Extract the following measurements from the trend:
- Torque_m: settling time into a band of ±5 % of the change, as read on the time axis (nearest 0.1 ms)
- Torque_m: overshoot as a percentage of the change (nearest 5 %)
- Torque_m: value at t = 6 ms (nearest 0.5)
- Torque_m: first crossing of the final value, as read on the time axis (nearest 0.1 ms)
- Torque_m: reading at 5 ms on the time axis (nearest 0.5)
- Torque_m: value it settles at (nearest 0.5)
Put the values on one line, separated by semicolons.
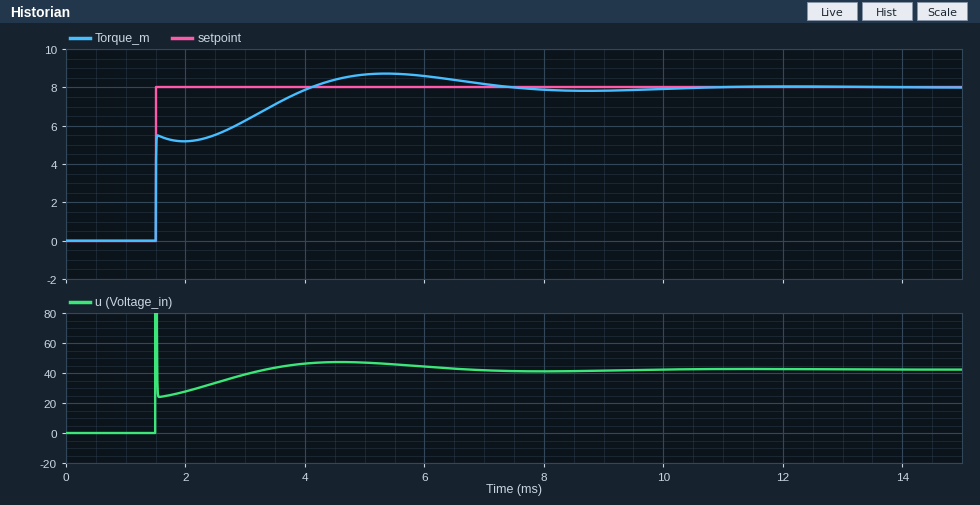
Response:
6.5 ms; 10 %; 8.5; 4.1 ms; 8.5; 8.0
